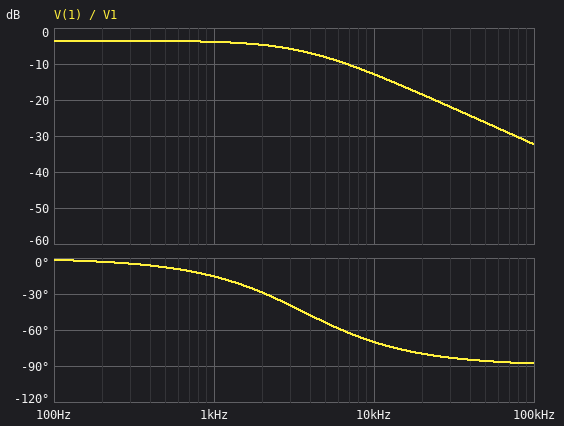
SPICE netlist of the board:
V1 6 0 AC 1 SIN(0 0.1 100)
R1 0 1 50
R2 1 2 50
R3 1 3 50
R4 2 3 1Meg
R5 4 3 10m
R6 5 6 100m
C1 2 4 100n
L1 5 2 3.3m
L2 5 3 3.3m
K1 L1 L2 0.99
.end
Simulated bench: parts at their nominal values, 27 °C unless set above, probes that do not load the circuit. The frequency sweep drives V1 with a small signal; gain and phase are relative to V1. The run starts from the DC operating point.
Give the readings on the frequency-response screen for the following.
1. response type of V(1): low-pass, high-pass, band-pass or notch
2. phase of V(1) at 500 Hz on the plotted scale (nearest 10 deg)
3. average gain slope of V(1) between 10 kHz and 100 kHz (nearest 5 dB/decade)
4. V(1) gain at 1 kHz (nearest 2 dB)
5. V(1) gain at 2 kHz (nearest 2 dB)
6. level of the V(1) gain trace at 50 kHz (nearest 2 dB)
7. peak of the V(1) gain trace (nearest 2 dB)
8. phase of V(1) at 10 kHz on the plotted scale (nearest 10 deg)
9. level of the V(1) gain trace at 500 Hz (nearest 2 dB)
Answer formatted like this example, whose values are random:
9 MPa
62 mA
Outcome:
low-pass
-10 deg
-20 dB/decade
-4 dB
-4 dB
-26 dB
-4 dB
-70 deg
-4 dB
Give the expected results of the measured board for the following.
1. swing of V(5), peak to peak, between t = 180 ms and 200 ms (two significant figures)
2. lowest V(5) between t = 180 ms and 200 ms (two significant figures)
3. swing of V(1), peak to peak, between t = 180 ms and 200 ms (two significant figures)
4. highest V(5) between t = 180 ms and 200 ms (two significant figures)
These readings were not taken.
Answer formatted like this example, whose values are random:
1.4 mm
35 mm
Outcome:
200 mV
-100 mV
130 mV
100 mV
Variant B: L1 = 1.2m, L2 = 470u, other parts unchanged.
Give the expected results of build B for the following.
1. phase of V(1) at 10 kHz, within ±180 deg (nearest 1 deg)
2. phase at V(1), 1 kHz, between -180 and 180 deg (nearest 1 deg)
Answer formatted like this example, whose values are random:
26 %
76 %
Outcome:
-33 deg
-4 deg
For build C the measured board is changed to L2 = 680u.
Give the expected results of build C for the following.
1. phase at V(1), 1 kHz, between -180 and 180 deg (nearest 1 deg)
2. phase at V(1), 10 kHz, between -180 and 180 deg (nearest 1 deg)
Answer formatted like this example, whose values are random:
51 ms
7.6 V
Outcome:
-8 deg
-28 deg
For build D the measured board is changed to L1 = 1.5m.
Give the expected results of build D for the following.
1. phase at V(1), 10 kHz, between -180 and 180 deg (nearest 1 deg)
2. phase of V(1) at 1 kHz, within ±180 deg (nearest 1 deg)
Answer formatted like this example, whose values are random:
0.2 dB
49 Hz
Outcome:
-53 deg
-11 deg
